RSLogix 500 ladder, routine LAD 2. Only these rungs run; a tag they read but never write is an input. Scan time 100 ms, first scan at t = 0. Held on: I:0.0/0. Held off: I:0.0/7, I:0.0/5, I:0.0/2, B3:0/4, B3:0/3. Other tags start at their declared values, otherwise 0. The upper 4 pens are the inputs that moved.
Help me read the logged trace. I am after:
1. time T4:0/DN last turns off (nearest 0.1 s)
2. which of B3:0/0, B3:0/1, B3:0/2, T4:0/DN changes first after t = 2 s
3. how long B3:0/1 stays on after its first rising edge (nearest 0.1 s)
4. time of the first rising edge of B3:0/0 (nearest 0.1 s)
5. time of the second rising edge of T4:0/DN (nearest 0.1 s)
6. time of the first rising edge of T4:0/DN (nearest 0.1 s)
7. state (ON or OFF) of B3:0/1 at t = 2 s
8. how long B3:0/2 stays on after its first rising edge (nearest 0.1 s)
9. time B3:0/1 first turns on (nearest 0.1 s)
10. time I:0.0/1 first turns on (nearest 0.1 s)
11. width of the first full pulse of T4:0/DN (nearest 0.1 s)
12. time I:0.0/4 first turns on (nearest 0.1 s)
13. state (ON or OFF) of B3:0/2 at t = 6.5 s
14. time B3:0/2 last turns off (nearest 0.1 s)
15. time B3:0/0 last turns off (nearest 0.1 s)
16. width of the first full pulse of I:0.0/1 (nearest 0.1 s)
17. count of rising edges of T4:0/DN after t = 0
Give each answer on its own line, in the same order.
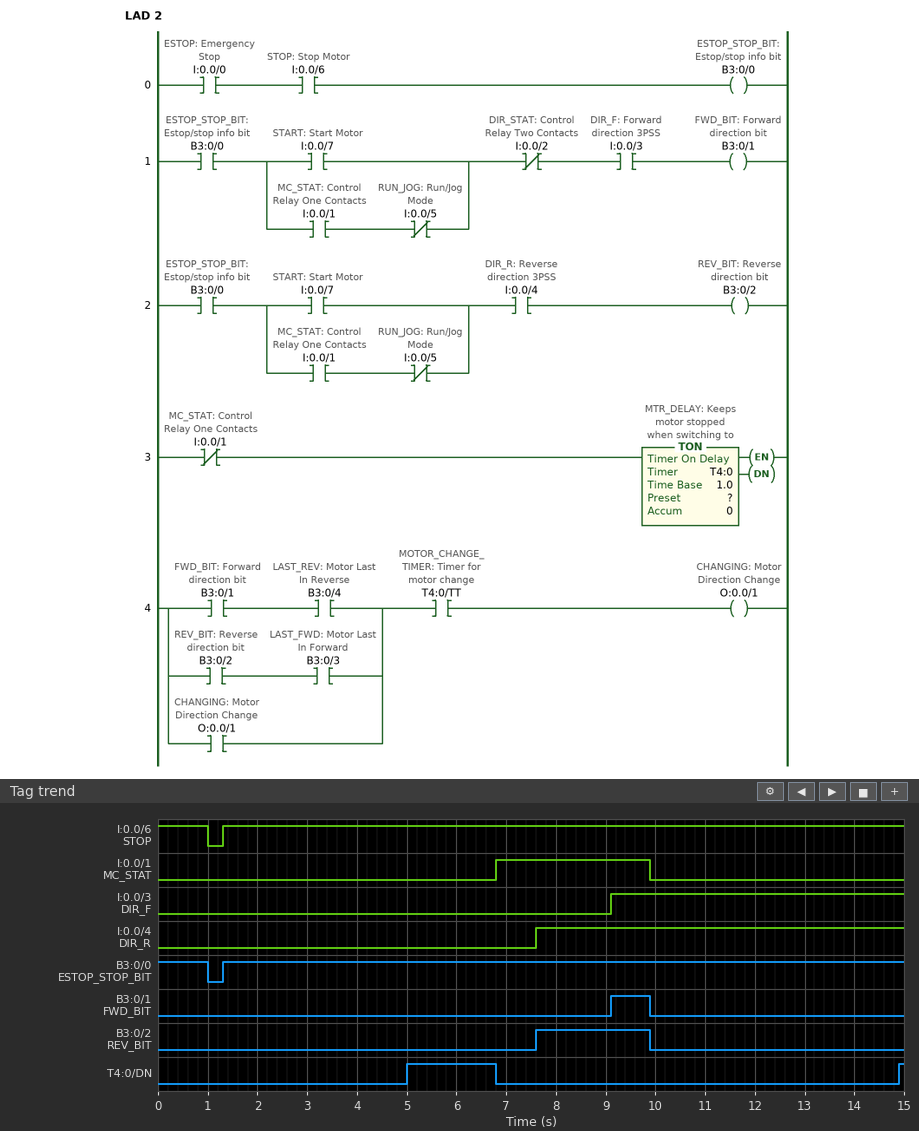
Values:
6.8 s
T4:0/DN
0.8 s
1.3 s
14.9 s
5.0 s
OFF
2.3 s
9.1 s
6.8 s
1.8 s
7.6 s
OFF
9.9 s
1.0 s
3.1 s
2
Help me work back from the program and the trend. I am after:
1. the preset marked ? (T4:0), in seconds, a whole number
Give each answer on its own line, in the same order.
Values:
5 s
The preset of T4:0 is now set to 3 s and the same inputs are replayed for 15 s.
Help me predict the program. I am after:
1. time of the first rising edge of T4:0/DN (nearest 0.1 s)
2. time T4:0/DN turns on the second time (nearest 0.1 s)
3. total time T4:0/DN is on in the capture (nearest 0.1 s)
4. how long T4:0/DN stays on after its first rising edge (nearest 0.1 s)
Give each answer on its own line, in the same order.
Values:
3.0 s
12.9 s
5.9 s
3.8 s
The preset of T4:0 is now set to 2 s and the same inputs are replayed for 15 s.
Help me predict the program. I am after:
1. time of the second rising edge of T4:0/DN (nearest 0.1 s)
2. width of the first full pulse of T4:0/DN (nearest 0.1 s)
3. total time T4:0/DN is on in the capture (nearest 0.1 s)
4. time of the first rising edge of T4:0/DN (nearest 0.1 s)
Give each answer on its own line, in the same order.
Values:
11.9 s
4.8 s
7.9 s
2.0 s
